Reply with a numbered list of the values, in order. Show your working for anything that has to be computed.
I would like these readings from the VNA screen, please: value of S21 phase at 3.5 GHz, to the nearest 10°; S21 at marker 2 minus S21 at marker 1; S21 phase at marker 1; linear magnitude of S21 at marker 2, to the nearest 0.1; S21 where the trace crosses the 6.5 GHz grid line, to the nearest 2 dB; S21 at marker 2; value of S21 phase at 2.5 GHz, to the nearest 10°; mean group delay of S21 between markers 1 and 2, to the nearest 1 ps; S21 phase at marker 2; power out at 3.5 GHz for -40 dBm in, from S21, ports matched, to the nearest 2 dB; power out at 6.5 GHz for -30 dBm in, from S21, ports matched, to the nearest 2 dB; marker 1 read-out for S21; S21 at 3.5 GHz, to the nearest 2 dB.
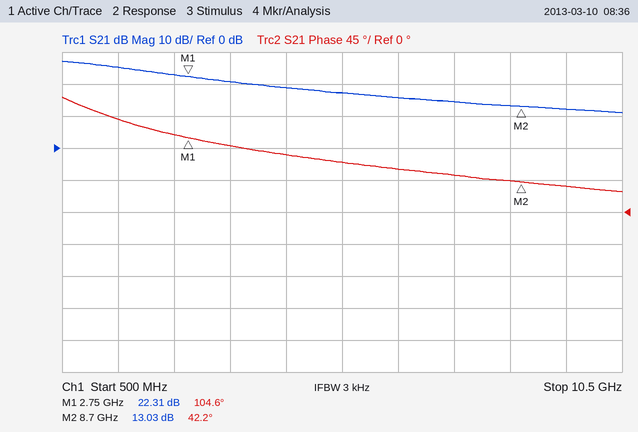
1. 90°
2. 13.03 − (22.31) = -9.28 dB
3. 104.6°
4. 10^(13.03/20) ≈ 4.5
5. 16 dB
6. 13.03 dB
7. 110°
8. −(42.2° − (104.6°))/(360° × 5.95 GHz) ≈ 29 ps
9. 42.2°
10. -40 dBm + (20 dB) = -20 dBm
11. -30 dBm + (16 dB) = -14 dBm
12. 22.31 dB
13. 20 dB
